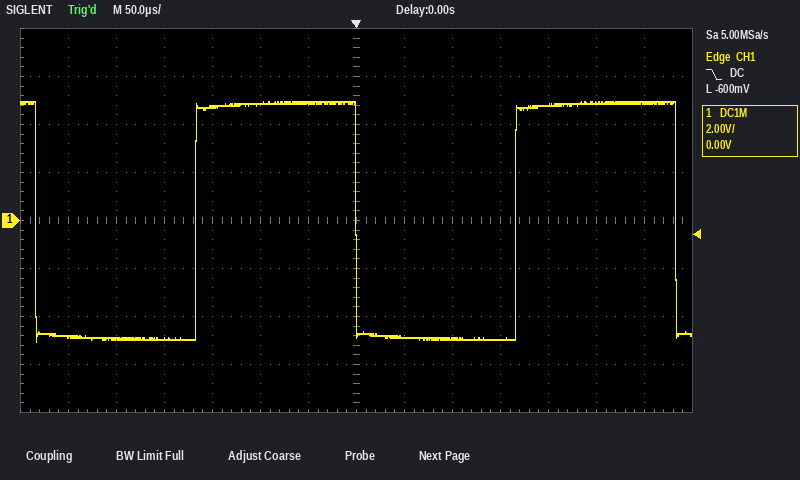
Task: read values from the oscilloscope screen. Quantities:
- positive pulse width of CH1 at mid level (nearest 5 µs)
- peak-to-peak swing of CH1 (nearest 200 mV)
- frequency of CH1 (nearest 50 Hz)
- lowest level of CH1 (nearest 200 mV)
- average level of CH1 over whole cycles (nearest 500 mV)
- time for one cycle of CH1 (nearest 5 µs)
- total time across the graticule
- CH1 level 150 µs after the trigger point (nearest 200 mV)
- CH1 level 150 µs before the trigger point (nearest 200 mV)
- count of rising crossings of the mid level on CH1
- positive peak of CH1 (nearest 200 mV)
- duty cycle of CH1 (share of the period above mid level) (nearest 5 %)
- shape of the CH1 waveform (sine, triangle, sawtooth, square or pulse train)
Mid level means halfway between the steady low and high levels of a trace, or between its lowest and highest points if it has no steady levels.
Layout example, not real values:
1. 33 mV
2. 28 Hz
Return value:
1. 165 µs
2. 10.0 V
3. 3.00 kHz
4. -5.0 V
5. 0.0 V
6. 335 µs
7. 700 µs
8. -5.0 V
9. 4.8 V
10. 2
11. 5.0 V
12. 50 %
13. square
